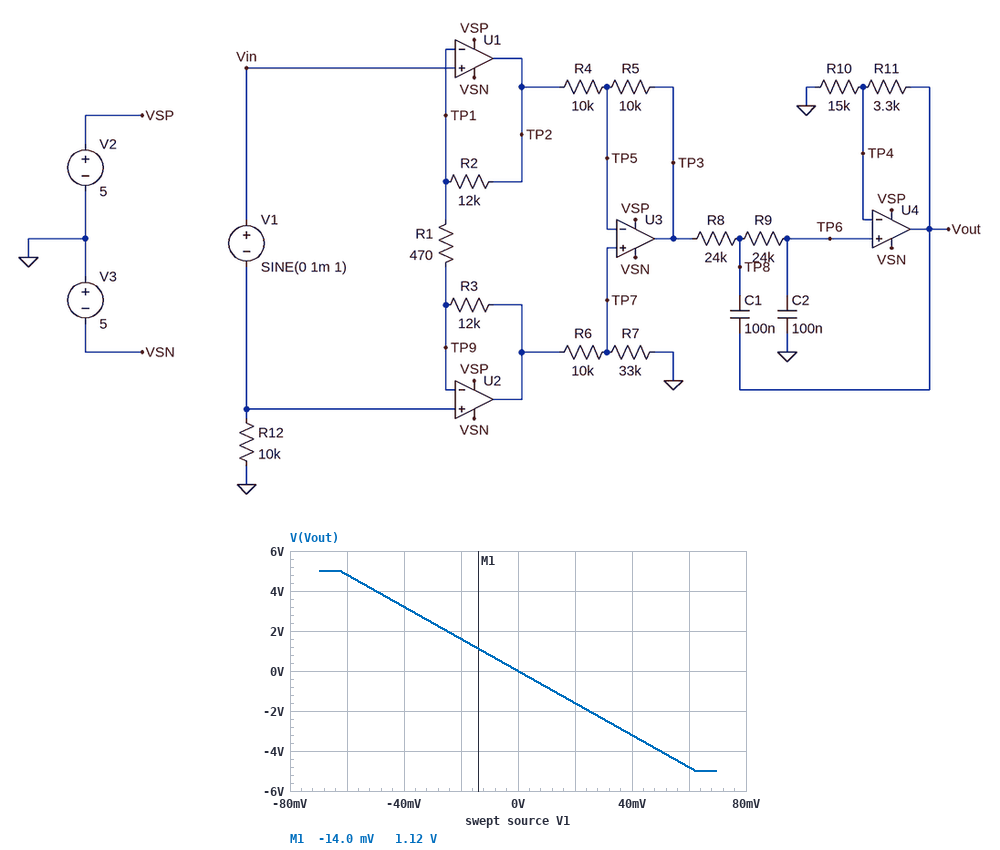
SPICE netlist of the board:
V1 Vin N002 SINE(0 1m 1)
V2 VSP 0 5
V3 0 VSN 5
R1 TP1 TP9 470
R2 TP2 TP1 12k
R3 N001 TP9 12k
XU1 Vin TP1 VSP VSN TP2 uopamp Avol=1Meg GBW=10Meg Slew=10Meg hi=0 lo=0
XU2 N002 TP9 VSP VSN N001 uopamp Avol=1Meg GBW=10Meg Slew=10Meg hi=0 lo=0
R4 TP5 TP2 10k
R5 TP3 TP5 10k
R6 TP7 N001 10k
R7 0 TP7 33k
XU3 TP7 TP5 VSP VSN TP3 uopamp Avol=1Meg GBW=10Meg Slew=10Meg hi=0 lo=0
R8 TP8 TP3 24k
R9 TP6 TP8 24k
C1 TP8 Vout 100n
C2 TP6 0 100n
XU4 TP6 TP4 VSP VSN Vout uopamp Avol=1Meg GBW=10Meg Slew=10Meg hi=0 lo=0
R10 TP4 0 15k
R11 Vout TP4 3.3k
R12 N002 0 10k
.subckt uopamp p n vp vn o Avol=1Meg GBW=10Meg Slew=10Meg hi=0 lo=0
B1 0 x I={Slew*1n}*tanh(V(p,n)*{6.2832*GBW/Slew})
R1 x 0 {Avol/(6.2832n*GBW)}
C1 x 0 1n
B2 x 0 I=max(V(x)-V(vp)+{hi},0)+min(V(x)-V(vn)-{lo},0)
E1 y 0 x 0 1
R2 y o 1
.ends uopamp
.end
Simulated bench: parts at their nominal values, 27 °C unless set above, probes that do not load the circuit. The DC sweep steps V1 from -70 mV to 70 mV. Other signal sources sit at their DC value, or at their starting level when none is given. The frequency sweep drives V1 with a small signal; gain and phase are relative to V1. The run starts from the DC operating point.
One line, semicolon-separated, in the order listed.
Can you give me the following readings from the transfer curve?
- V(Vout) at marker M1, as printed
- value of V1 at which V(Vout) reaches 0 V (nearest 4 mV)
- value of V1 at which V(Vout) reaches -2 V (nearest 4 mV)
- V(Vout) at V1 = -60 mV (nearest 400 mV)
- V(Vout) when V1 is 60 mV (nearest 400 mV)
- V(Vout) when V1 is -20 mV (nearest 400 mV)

1.12 V; 0 V; 24 mV; 4.8 V; -4.8 V; 1.6 V
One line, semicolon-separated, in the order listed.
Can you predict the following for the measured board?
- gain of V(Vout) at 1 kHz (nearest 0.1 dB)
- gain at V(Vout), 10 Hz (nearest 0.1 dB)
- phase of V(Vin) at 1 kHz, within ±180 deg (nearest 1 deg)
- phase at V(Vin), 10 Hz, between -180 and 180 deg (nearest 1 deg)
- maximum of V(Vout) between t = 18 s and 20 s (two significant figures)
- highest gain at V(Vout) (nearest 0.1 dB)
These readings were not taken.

-9.1 dB; 38.0 dB; 0 deg; 0 deg; 80 mV; 38.1 dB
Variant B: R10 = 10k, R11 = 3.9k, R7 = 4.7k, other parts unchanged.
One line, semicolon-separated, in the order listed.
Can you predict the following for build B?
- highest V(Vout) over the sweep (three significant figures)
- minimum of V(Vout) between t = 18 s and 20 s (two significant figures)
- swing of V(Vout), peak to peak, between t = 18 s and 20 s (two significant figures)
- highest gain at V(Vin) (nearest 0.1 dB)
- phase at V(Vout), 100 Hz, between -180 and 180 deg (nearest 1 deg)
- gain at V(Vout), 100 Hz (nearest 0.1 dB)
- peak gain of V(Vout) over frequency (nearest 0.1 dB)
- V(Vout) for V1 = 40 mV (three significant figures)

4.17 V; -60 mV; 120 mV; 0 dB; 62 deg; 26.7 dB; 35.5 dB; -2.38 V
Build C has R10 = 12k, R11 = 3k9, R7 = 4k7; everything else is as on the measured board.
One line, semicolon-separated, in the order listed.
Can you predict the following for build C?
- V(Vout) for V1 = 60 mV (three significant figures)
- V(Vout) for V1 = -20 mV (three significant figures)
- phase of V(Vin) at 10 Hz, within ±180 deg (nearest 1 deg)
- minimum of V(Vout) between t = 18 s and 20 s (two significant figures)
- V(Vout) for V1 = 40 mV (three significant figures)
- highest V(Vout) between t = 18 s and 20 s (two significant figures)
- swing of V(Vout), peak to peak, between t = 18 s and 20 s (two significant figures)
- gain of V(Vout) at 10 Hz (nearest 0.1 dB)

-3.41 V; 1.14 V; 0 deg; -57 mV; -2.27 V; 57 mV; 110 mV; 35.0 dB
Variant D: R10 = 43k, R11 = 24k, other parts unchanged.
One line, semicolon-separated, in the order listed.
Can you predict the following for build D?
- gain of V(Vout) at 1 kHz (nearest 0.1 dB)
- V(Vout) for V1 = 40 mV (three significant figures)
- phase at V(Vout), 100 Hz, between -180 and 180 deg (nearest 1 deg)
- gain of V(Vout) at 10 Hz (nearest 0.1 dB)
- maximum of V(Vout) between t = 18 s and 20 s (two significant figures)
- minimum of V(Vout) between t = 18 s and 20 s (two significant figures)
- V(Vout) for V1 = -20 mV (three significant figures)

-6.9 dB; -4.10 V; 60 deg; 40.2 dB; 100 mV; -100 mV; 2.05 V
